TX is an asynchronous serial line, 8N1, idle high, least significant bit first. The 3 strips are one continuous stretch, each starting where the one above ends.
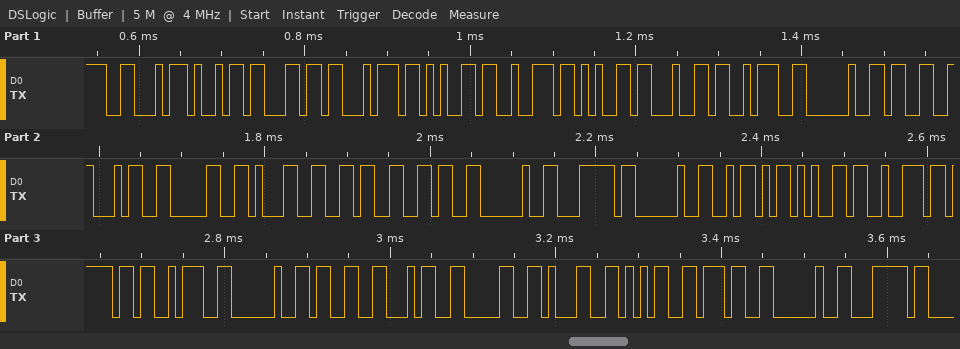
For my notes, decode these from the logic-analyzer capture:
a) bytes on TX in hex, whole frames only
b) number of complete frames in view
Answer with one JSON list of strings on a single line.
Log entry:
["46 69 6C 74 65 72 65 64 3A 20 33 34 30 31 36 36 20 7C 20 5A 65 72 6F 3A 20 33 34 30 31 35 37 20 7C", "33"]
